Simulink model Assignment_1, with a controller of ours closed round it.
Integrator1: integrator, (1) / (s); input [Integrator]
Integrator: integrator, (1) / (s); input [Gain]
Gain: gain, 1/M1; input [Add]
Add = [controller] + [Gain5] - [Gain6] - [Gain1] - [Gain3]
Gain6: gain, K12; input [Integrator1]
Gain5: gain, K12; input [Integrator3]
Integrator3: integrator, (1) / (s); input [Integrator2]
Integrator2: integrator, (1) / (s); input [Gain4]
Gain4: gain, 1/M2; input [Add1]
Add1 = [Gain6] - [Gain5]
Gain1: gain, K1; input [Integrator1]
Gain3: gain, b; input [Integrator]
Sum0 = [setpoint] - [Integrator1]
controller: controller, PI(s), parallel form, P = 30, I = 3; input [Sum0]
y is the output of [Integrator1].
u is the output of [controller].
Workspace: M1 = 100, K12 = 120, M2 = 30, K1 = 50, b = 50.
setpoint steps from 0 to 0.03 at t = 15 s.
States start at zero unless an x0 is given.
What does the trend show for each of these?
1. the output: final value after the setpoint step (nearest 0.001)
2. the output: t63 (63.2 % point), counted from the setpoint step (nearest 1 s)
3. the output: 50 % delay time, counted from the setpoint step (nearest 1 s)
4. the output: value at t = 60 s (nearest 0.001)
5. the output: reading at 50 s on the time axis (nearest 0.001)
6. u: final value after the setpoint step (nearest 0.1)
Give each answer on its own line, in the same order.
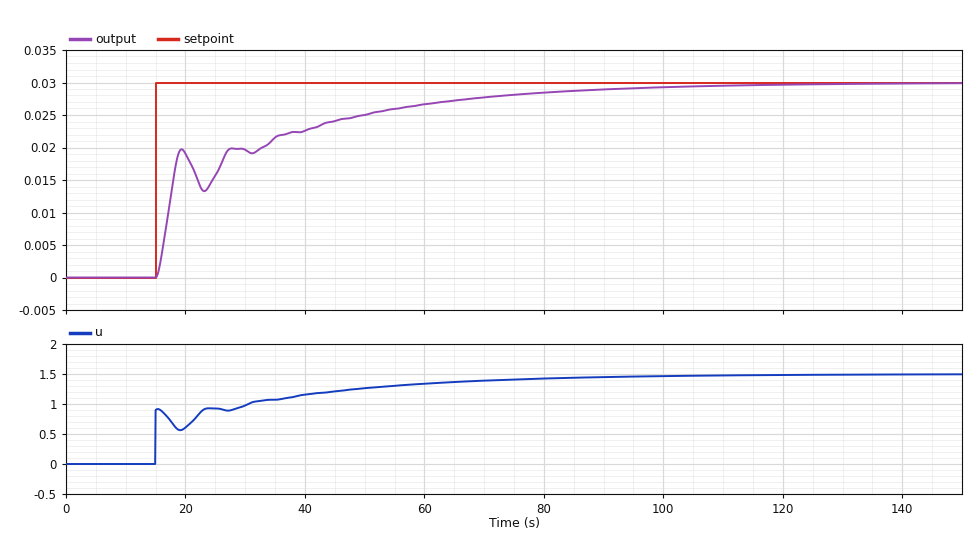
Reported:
0.030
4 s
3 s
0.027
0.025
1.5
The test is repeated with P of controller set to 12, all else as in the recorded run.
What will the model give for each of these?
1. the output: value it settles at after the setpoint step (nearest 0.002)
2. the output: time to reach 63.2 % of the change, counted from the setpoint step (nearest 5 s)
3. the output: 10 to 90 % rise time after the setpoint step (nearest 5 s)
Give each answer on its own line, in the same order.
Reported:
0.030
15 s
40 s
